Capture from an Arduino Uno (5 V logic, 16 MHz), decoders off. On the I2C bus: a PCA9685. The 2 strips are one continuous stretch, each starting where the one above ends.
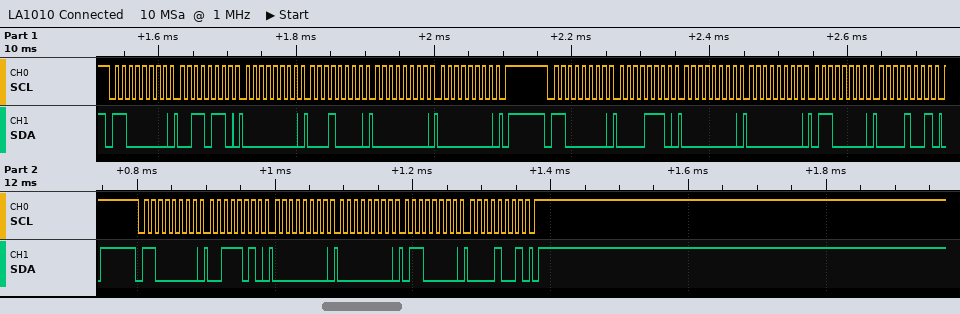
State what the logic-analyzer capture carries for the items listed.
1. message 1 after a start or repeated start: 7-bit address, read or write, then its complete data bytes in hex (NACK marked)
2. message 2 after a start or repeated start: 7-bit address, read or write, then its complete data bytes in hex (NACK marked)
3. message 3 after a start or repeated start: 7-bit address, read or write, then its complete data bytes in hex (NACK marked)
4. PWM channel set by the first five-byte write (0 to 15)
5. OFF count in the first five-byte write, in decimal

0x60 write: 36 00 10 00 00
0x60 write: 0E 00 00 60 09
0x60 write: 3A 00 00 60 09
12
0
